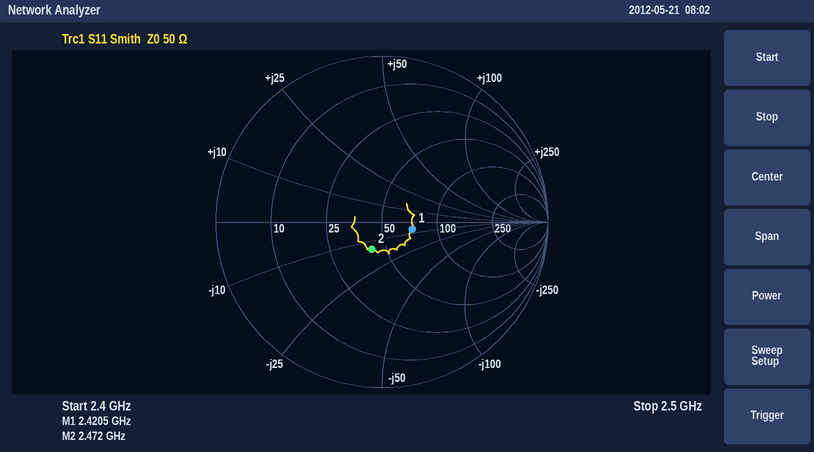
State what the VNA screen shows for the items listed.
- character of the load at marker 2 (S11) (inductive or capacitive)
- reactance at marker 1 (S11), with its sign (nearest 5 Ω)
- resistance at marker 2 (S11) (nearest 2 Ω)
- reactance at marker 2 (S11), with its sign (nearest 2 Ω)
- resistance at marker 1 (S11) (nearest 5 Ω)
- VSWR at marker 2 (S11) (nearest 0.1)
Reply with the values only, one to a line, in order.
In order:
capacitive
-5 Ω
42 Ω
-14 Ω
70 Ω
1.4
